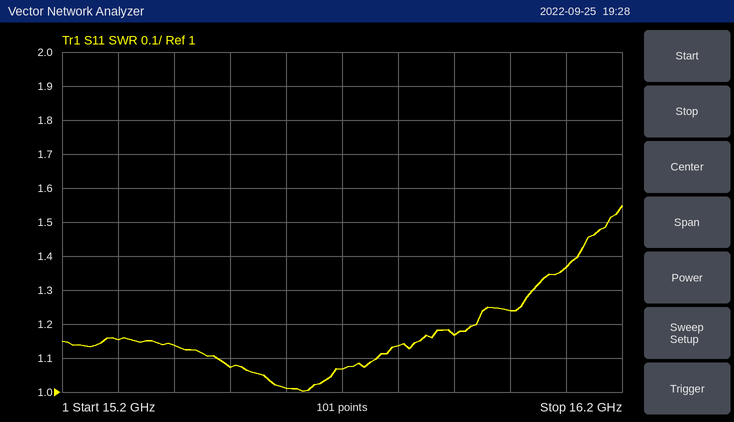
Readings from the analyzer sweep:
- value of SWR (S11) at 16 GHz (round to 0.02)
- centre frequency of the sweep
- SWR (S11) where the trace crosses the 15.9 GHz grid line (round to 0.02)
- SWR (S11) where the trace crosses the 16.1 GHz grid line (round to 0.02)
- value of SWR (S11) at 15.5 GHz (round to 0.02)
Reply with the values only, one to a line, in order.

1.24
15.7 GHz
1.16
1.36
1.08
